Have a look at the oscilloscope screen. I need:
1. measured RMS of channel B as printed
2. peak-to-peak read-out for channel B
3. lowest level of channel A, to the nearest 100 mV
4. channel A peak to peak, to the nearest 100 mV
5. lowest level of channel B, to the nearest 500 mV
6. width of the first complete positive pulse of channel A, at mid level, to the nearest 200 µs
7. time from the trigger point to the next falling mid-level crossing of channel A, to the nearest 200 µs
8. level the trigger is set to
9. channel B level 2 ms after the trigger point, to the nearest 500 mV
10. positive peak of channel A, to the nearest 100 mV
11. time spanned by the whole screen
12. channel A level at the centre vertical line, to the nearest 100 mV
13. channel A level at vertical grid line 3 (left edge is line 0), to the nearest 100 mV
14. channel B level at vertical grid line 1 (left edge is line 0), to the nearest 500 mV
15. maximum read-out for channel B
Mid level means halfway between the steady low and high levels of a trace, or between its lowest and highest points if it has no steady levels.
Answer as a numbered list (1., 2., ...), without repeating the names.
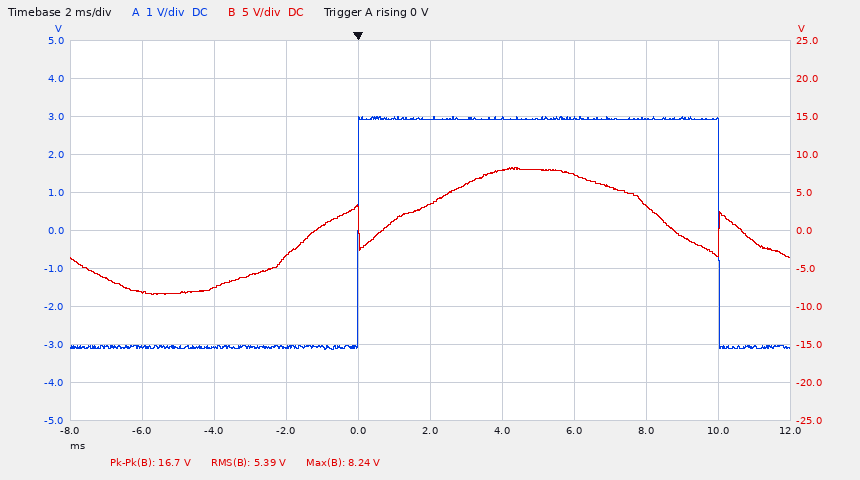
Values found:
1. 5.39 V
2. 16.7 V
3. -3.1 V
4. 6.1 V
5. -8.5 V
6. 10.0 ms
7. 10.0 ms
8. 0 V
9. 3.5 V
10. 3.0 V
11. 20 ms
12. 2.9 V
13. -3.1 V
14. -8.0 V
15. 8.24 V
